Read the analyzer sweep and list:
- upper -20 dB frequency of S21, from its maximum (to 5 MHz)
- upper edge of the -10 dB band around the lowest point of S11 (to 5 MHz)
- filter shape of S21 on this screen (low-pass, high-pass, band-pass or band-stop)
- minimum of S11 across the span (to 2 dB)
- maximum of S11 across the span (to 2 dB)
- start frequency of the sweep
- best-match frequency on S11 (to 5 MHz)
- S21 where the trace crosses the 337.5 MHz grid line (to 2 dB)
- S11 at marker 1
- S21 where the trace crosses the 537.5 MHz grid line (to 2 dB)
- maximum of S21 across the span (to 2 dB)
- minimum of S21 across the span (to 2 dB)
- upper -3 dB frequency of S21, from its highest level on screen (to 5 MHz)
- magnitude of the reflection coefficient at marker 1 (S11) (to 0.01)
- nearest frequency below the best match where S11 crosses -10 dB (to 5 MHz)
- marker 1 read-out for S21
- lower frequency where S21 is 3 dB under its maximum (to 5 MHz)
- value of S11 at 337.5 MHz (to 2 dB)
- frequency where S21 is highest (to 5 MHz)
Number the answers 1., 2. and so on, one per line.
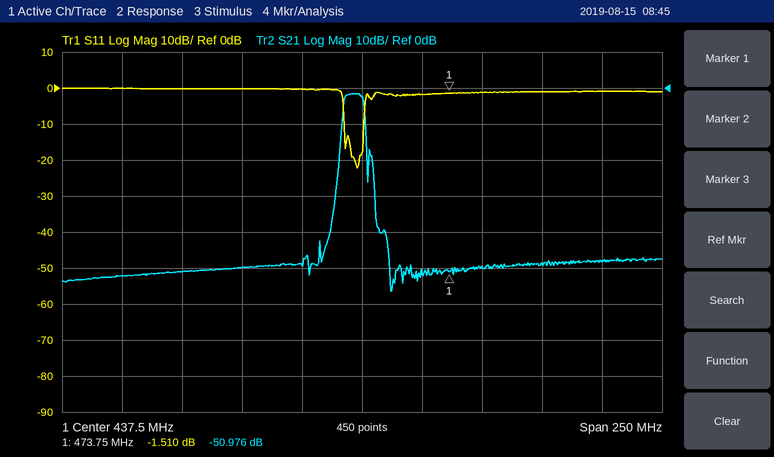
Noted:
1. 440 MHz
2. 440 MHz
3. band-pass
4. -22 dB
5. 0 dB
6. 312.5 MHz
7. 435 MHz
8. -52 dB
9. -1.510 dB
10. -48 dB
11. -2 dB
12. -56 dB
13. 440 MHz
14. 0.84
15. 430 MHz
16. -50.976 dB
17. 430 MHz
18. 0 dB
19. 435 MHz
